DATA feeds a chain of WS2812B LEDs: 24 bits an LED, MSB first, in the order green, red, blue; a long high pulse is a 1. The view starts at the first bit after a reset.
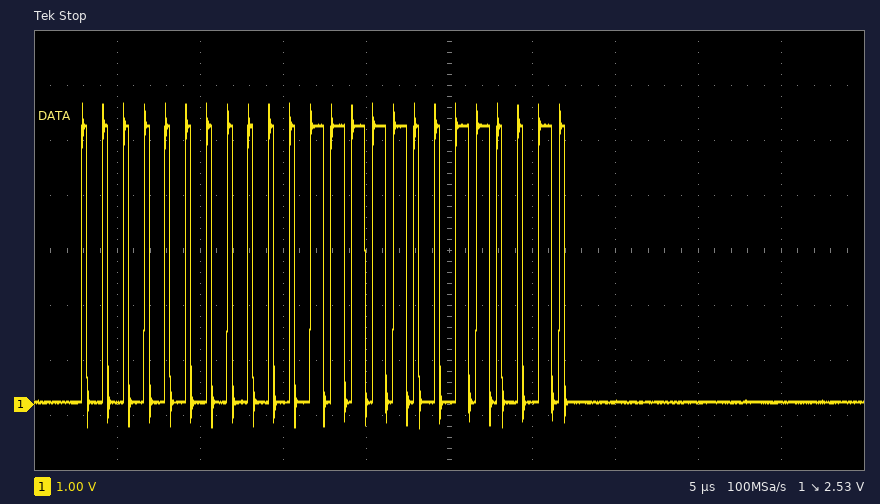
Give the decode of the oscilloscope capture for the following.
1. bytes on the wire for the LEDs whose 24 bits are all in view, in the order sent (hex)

00 1F 32
